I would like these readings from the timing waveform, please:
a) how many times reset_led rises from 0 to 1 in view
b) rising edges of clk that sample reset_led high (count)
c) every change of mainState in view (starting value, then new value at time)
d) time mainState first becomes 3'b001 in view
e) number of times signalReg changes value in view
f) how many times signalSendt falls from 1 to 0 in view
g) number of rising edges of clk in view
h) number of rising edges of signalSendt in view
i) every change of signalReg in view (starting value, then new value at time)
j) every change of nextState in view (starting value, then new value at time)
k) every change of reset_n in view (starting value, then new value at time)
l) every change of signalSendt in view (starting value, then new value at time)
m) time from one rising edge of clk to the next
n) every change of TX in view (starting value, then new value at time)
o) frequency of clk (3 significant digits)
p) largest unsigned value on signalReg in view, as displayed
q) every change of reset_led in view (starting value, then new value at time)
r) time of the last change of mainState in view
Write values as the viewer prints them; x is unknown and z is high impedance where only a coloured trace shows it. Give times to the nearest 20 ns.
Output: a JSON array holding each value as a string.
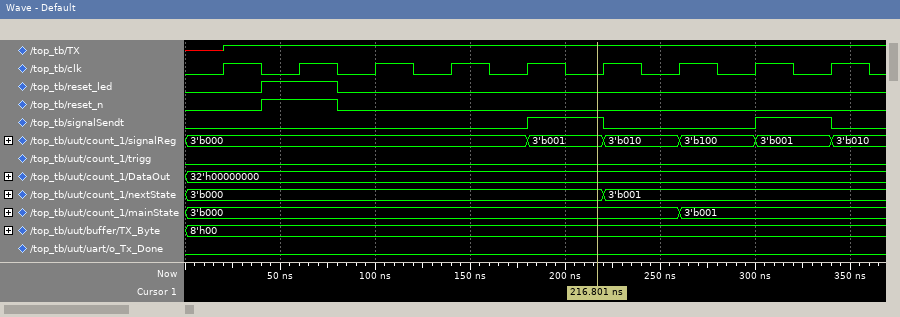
["1", "1", "3'b000, 3'b001 at 260 ns", "260 ns", "5", "2", "9", "2", "3'b000, 3'b001 at 180 ns, 3'b010 at 220 ns, 3'b100 at 260 ns, 3'b001 at 300 ns, 3'b010 at 340 ns", "3'b000, 3'b001 at 220 ns", "0, 1 at 40 ns, 0 at 80 ns", "0, 1 at 180 ns, 0 at 220 ns, 1 at 300 ns, 0 at 340 ns", "40 ns", "x, 1 at 20 ns", "25.0 MHz", "3'b100", "0, 1 at 40 ns, 0 at 80 ns", "260 ns"]
